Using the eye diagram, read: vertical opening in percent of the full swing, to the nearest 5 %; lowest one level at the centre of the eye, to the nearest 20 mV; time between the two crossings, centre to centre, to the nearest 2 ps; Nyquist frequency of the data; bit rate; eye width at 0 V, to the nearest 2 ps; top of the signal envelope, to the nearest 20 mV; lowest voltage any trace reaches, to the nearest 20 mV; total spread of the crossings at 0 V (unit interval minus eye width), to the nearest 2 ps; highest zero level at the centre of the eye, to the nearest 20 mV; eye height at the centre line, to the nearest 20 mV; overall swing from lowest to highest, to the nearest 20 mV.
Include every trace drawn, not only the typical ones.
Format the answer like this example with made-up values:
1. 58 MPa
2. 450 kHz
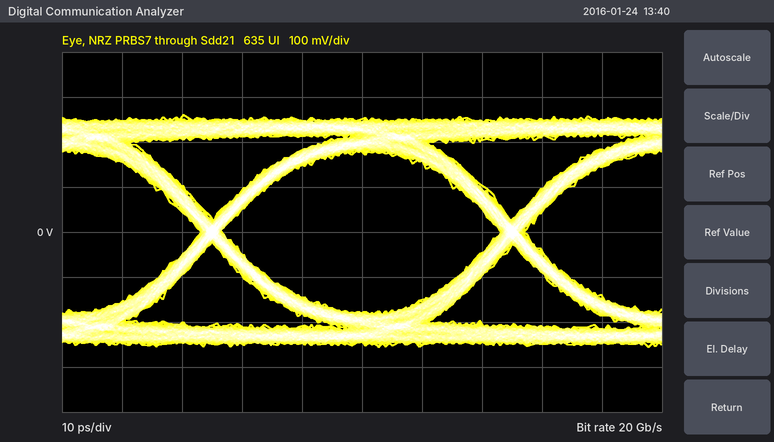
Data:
1. 70 %
2. 180 mV
3. 50 ps
4. 10 GHz
5. 20 Gb/s
6. 46 ps
7. 260 mV
8. -260 mV
9. 4 ps
10. -180 mV
11. 360 mV
12. 520 mV
